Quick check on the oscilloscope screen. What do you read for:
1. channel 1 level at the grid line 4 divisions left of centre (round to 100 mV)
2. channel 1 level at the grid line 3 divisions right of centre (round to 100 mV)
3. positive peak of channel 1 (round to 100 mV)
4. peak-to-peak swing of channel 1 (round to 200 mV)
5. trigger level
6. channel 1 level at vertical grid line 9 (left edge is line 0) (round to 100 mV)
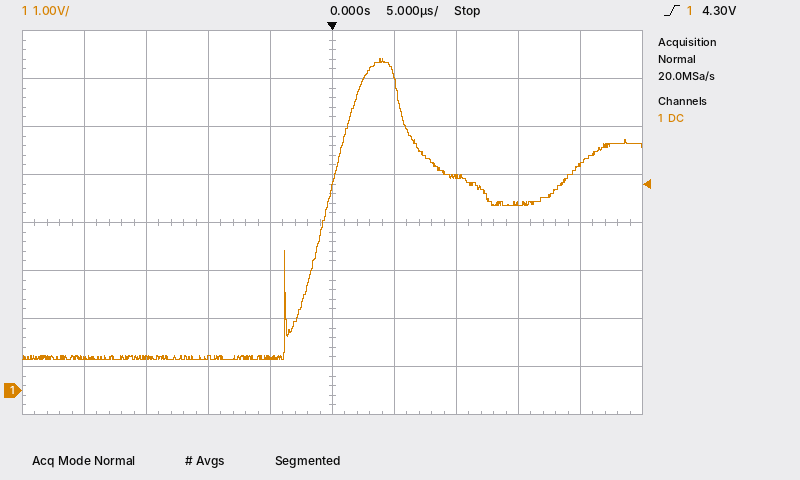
700 mV
3.9 V
6.9 V
6.2 V
4.30 V
4.7 V
